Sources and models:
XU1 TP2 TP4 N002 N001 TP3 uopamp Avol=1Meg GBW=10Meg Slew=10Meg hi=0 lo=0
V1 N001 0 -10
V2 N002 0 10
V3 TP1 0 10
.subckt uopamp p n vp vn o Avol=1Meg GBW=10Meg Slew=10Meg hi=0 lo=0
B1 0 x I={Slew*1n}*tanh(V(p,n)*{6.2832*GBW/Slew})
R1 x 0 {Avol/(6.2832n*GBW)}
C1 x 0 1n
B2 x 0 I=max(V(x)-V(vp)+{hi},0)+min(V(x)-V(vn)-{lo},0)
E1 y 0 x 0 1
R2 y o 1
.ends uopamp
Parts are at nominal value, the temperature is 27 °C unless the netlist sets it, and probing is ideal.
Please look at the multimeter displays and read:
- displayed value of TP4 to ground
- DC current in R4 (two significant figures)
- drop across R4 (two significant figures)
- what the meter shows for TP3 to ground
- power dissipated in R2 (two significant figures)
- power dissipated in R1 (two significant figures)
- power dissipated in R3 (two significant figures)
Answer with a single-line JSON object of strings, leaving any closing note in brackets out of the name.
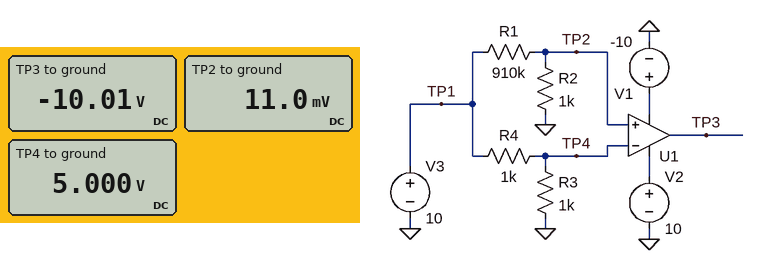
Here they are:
{"displayed value of TP4 to ground": "5.000 V", "DC current in R4": "5.0 mA", "drop across R4": "5.0 V", "what the meter shows for TP3 to ground": "-10.01 V", "power dissipated in R2": "120 nW", "power dissipated in R1": "110 µW", "power dissipated in R3": "25 mW"}
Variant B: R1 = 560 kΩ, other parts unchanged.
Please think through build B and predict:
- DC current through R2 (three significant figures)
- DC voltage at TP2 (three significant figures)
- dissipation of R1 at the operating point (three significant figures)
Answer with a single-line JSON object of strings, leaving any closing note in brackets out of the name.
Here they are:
{"DC current through R2": "17.8 µA", "DC voltage at TP2": "17.8 mV", "dissipation of R1 at the operating point": "178 µW"}
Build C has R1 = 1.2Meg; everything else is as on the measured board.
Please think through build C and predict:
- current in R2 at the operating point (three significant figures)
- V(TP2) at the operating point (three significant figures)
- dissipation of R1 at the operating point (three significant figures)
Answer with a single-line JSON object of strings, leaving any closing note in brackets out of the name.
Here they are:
{"current in R2 at the operating point": "8.33 µA", "V(TP2) at the operating point": "8.33 mV", "dissipation of R1 at the operating point": "83.2 µW"}
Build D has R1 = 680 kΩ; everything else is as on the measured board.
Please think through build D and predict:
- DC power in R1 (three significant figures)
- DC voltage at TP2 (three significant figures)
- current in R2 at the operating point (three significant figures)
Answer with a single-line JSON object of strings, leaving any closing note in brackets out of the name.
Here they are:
{"DC power in R1": "147 µW", "DC voltage at TP2": "14.7 mV", "current in R2 at the operating point": "14.7 µA"}
